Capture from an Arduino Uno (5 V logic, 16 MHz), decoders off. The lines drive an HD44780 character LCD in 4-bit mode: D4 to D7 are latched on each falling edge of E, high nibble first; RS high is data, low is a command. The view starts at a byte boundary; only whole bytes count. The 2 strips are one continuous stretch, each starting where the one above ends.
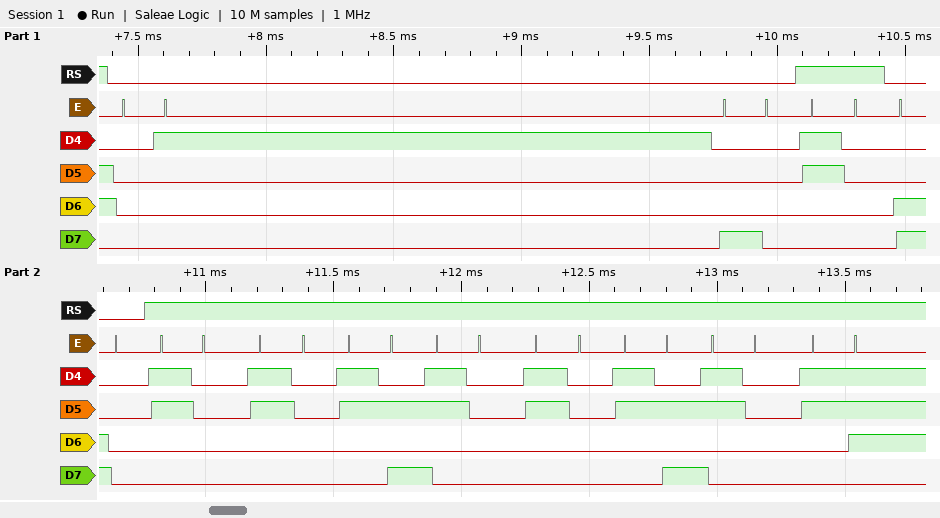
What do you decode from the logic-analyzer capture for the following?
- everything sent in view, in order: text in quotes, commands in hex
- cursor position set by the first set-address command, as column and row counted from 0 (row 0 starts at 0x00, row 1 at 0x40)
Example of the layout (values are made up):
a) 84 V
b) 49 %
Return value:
a) 0x01 0x80 "0" 0xC0 "00:00:07"
b) column 0, row 0
